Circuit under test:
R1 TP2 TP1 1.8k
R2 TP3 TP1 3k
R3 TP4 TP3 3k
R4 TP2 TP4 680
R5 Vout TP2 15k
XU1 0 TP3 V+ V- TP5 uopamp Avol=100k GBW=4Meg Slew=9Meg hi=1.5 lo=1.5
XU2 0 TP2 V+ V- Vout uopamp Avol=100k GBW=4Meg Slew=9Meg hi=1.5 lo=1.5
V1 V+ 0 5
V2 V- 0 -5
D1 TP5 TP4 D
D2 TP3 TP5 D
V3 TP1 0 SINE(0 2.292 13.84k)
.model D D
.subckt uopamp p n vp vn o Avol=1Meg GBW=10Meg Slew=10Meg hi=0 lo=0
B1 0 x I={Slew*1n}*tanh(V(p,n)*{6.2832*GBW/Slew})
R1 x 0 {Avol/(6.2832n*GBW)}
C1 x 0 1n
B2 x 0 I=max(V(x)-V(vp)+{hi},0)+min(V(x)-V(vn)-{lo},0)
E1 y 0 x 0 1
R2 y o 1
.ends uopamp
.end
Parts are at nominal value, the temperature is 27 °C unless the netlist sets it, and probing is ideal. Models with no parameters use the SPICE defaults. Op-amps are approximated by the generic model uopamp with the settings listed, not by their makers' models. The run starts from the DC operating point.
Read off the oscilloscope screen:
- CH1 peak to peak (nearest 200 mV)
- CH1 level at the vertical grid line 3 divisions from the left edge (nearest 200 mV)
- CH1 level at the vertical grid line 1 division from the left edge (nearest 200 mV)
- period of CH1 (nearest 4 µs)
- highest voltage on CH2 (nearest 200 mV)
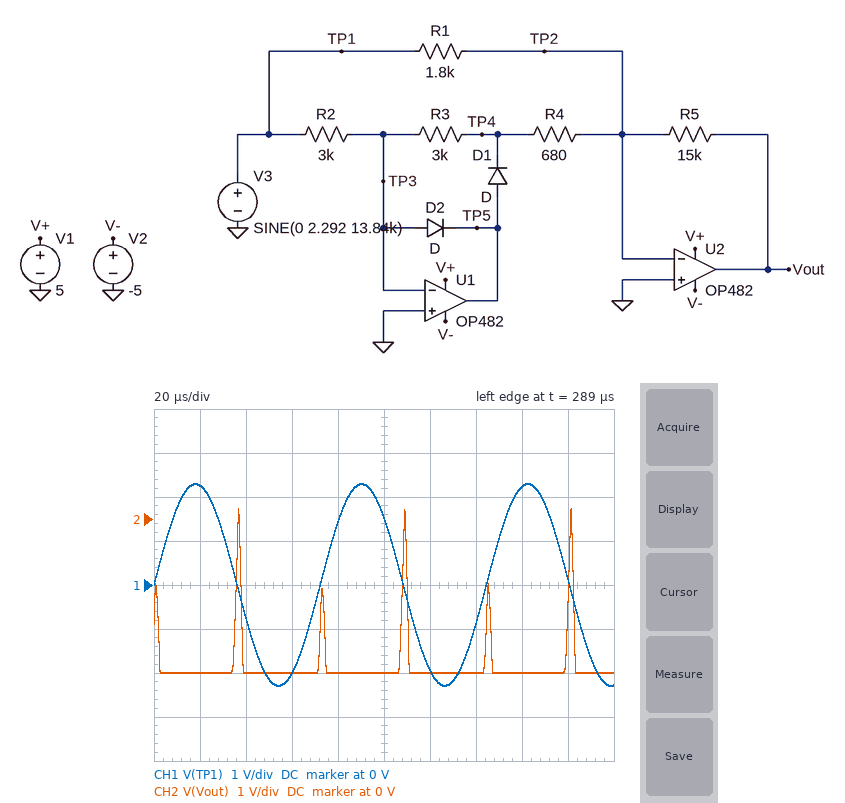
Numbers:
4.6 V
-2.0 V
2.2 V
72 µs
200 mV
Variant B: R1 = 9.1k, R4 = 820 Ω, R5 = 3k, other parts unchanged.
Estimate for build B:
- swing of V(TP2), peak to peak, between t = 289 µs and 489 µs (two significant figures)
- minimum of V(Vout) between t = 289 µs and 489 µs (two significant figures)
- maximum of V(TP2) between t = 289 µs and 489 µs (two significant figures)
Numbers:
850 mV
-3.5 V
830 mV
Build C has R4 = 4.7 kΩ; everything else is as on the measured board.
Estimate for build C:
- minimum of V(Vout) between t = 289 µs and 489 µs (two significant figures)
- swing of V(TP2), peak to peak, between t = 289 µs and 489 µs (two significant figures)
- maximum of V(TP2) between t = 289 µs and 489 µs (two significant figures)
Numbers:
-3.5 V
2.0 V
1.4 V
